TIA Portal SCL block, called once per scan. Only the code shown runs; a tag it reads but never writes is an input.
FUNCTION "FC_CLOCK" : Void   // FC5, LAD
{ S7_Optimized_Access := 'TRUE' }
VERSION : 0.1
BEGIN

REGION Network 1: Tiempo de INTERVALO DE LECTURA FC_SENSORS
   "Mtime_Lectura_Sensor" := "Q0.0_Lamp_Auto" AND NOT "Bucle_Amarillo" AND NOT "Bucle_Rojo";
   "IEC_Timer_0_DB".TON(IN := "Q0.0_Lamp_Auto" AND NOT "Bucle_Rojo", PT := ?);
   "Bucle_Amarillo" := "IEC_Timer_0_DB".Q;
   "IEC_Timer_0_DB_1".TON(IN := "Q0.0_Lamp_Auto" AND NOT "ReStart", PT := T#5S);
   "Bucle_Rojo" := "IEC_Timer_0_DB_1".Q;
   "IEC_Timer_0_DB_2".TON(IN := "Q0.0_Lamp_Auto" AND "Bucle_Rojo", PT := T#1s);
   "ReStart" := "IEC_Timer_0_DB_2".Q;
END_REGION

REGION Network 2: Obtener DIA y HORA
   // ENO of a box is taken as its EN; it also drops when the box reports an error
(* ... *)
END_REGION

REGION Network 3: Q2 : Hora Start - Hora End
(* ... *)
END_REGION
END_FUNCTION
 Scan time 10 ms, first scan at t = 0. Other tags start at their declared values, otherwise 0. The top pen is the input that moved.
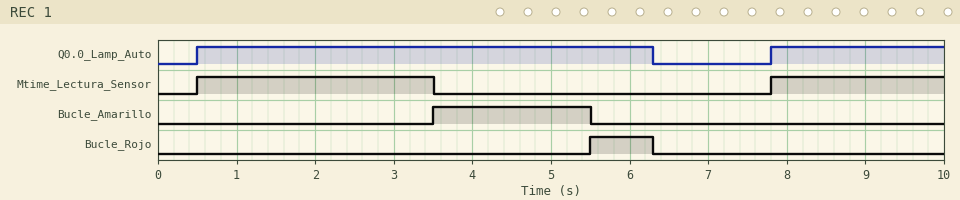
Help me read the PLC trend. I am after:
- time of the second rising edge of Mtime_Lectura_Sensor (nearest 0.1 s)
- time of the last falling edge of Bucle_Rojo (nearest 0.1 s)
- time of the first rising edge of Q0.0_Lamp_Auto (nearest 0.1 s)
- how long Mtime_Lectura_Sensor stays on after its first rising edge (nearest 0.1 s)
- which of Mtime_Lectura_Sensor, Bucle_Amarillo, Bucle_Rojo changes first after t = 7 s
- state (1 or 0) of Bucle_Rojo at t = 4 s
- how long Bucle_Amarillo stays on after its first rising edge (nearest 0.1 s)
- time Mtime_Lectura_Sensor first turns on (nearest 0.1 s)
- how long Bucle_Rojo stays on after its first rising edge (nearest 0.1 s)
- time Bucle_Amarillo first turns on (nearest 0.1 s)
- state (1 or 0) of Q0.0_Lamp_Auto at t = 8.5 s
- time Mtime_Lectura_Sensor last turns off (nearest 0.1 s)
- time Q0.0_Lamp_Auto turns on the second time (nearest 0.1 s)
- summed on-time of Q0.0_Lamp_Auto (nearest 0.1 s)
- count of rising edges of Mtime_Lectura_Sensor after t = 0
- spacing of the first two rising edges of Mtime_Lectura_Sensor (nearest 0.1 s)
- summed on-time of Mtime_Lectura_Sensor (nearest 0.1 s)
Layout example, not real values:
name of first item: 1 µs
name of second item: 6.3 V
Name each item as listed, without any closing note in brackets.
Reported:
time of the second rising edge of Mtime_Lectura_Sensor: 7.8 s
time of the last falling edge of Bucle_Rojo: 6.3 s
time of the first rising edge of Q0.0_Lamp_Auto: 0.5 s
how long Mtime_Lectura_Sensor stays on after its first rising edge: 3.0 s
which of Mtime_Lectura_Sensor, Bucle_Amarillo, Bucle_Rojo changes first after t = 7 s: Mtime_Lectura_Sensor
state (1 or 0) of Bucle_Rojo at t = 4 s: 0
how long Bucle_Amarillo stays on after its first rising edge: 2.0 s
time Mtime_Lectura_Sensor first turns on: 0.5 s
how long Bucle_Rojo stays on after its first rising edge: 0.8 s
time Bucle_Amarillo first turns on: 3.5 s
state (1 or 0) of Q0.0_Lamp_Auto at t = 8.5 s: 1
time Mtime_Lectura_Sensor last turns off: 3.5 s
time Q0.0_Lamp_Auto turns on the second time: 7.8 s
summed on-time of Q0.0_Lamp_Auto: 8.0 s
count of rising edges of Mtime_Lectura_Sensor after t = 0: 2
spacing of the first two rising edges of Mtime_Lectura_Sensor: 7.3 s
summed on-time of Mtime_Lectura_Sensor: 5.2 s
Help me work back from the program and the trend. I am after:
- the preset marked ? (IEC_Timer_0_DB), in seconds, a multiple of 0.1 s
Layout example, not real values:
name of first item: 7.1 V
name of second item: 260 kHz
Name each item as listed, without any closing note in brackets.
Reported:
the preset marked ? (IEC_Timer_0_DB), in seconds, a multiple of 0.1 s: 3.0 s
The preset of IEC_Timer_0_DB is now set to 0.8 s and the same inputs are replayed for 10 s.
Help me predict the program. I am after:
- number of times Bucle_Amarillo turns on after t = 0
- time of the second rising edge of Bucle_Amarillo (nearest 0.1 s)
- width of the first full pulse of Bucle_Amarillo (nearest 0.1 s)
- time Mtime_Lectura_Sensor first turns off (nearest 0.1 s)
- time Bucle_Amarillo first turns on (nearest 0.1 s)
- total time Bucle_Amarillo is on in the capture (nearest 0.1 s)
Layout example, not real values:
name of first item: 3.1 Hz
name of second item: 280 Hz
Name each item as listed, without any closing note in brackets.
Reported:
number of times Bucle_Amarillo turns on after t = 0: 2
time of the second rising edge of Bucle_Amarillo: 8.6 s
width of the first full pulse of Bucle_Amarillo: 4.2 s
time Mtime_Lectura_Sensor first turns off: 1.3 s
time Bucle_Amarillo first turns on: 1.3 s
total time Bucle_Amarillo is on in the capture: 5.6 s
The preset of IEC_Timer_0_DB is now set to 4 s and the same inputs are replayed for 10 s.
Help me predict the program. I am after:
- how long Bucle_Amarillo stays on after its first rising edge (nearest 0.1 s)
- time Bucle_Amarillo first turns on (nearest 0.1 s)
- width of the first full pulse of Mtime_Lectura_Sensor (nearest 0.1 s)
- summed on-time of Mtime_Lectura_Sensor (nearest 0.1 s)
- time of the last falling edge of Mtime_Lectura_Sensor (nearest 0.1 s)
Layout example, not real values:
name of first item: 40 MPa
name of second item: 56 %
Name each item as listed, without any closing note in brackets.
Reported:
how long Bucle_Amarillo stays on after its first rising edge: 1.0 s
time Bucle_Amarillo first turns on: 4.5 s
width of the first full pulse of Mtime_Lectura_Sensor: 4.0 s
summed on-time of Mtime_Lectura_Sensor: 6.2 s
time of the last falling edge of Mtime_Lectura_Sensor: 4.5 s
